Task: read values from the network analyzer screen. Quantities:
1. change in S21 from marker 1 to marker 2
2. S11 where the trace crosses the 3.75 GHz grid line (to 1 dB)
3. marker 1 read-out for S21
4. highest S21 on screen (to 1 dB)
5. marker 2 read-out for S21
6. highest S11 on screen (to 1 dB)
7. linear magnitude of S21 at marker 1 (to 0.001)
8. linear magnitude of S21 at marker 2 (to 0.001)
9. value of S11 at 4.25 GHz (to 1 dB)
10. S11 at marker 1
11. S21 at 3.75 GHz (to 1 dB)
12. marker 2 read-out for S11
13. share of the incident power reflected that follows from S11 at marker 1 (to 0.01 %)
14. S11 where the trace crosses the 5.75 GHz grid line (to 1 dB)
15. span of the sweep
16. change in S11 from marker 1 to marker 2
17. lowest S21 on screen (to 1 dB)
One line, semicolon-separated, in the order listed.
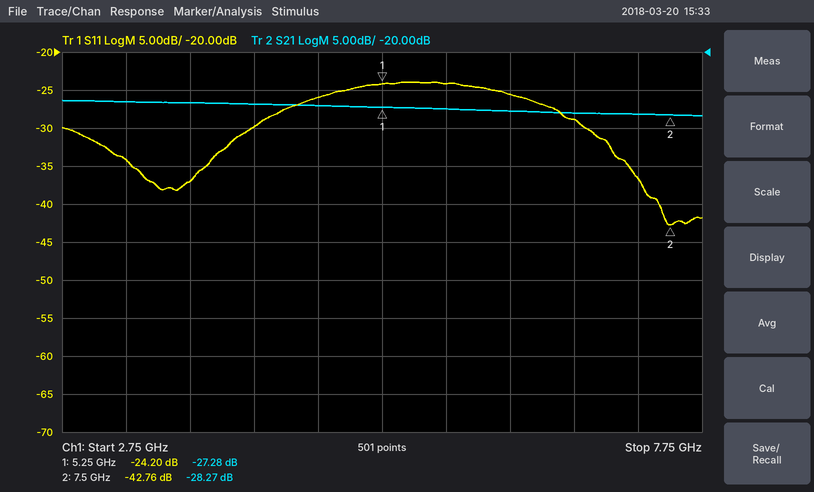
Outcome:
-0.99 dB; -37 dB; -27.28 dB; -26 dB; -28.27 dB; -24 dB; 0.043; 0.039; -30 dB; -24.20 dB; -27 dB; -42.76 dB; 0.38 %; -24 dB; 5 GHz; -18.56 dB; -28 dB
